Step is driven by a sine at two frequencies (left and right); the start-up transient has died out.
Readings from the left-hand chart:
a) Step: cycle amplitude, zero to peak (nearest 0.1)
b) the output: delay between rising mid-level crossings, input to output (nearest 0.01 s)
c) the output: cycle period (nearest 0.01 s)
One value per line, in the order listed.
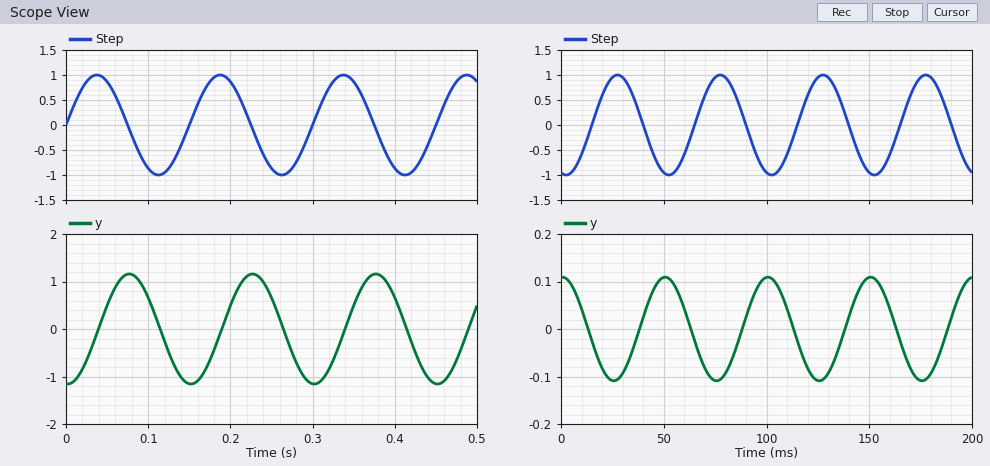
1.0
0.04 s
0.15 s
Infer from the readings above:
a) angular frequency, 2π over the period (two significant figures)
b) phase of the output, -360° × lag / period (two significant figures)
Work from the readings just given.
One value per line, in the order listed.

42 rad/s
-96°
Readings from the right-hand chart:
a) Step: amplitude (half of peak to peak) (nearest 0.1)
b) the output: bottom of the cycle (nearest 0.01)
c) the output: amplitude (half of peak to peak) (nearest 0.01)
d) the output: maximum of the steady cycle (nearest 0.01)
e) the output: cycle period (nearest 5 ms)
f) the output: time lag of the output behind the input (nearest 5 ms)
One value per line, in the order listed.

1.0
-0.11
0.11
0.11
50 ms
25 ms
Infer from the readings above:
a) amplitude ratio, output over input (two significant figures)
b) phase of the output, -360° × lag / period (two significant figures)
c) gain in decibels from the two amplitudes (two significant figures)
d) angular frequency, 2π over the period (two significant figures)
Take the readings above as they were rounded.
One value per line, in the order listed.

0.11
-180°
-19 dB
0.13 rad/ms
